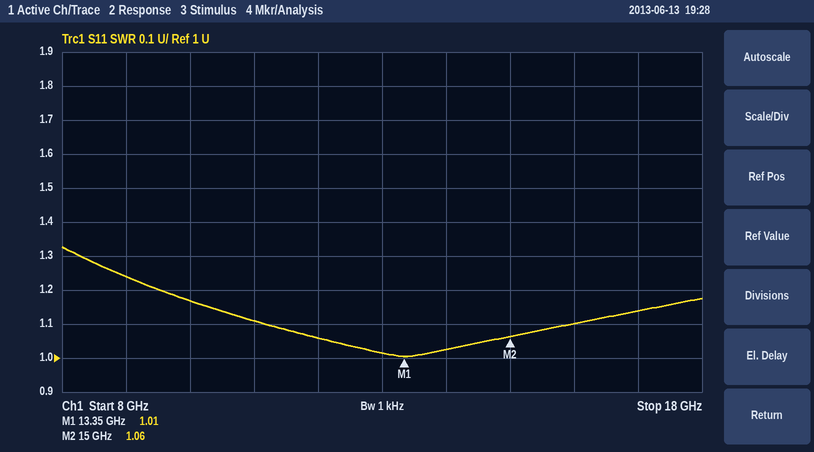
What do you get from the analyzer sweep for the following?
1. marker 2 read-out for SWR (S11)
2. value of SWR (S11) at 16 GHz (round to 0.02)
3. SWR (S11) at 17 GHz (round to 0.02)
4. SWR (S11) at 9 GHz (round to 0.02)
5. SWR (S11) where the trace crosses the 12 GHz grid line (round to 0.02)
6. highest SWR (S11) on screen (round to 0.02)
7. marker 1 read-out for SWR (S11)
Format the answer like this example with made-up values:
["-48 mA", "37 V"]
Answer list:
["1.06", "1.10", "1.14", "1.24", "1.06", "1.32", "1.01"]
